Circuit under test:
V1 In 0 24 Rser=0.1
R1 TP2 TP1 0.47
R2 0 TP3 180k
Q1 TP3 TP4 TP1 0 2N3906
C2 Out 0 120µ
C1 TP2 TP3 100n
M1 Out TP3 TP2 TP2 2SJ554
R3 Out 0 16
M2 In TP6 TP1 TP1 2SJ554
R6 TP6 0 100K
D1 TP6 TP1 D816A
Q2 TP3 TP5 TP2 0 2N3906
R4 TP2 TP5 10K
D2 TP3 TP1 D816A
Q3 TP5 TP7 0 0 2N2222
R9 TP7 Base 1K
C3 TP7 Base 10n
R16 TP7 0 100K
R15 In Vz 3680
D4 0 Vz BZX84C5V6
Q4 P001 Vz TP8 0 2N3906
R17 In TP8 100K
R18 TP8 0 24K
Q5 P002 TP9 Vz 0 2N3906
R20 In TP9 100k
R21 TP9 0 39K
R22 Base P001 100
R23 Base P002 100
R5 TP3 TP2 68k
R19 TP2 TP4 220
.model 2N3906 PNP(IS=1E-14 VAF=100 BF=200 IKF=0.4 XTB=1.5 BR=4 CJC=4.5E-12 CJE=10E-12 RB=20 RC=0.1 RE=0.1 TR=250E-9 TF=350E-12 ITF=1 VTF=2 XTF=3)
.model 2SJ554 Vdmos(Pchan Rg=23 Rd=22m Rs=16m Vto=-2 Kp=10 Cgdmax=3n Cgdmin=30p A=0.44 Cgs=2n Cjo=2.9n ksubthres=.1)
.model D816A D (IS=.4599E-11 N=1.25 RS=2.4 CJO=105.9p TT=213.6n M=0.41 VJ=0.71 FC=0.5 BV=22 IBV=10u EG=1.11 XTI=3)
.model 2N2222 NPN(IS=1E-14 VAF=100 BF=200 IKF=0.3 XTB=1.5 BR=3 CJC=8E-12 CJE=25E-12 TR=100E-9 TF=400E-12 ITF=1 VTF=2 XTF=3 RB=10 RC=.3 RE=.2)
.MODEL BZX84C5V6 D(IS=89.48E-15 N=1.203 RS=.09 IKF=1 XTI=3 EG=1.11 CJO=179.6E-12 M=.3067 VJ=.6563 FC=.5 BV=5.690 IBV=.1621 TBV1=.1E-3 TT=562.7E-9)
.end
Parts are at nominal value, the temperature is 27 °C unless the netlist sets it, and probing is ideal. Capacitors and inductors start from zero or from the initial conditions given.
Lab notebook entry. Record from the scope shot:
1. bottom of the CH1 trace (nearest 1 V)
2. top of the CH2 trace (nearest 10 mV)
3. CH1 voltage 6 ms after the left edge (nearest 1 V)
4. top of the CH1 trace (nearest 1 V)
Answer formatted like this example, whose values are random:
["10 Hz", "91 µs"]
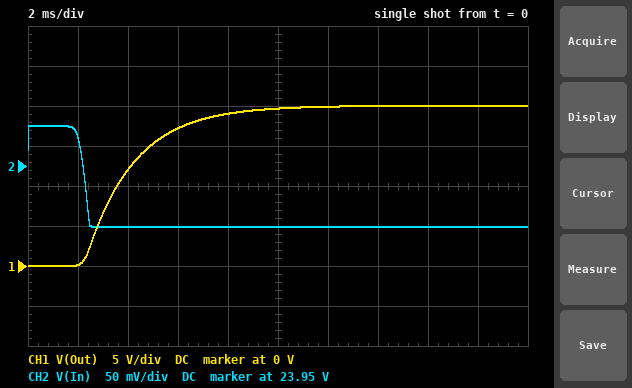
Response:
["0 V", "24.00 V", "17 V", "20 V"]
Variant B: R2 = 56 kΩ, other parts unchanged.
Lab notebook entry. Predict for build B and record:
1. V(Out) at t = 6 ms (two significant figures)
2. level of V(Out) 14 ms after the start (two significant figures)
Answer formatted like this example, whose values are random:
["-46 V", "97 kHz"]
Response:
["20 V", "21 V"]
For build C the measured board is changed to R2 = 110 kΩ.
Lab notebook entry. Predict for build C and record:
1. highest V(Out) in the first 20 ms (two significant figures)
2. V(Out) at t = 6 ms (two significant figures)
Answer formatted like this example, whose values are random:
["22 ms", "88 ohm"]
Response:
["21 V", "19 V"]
